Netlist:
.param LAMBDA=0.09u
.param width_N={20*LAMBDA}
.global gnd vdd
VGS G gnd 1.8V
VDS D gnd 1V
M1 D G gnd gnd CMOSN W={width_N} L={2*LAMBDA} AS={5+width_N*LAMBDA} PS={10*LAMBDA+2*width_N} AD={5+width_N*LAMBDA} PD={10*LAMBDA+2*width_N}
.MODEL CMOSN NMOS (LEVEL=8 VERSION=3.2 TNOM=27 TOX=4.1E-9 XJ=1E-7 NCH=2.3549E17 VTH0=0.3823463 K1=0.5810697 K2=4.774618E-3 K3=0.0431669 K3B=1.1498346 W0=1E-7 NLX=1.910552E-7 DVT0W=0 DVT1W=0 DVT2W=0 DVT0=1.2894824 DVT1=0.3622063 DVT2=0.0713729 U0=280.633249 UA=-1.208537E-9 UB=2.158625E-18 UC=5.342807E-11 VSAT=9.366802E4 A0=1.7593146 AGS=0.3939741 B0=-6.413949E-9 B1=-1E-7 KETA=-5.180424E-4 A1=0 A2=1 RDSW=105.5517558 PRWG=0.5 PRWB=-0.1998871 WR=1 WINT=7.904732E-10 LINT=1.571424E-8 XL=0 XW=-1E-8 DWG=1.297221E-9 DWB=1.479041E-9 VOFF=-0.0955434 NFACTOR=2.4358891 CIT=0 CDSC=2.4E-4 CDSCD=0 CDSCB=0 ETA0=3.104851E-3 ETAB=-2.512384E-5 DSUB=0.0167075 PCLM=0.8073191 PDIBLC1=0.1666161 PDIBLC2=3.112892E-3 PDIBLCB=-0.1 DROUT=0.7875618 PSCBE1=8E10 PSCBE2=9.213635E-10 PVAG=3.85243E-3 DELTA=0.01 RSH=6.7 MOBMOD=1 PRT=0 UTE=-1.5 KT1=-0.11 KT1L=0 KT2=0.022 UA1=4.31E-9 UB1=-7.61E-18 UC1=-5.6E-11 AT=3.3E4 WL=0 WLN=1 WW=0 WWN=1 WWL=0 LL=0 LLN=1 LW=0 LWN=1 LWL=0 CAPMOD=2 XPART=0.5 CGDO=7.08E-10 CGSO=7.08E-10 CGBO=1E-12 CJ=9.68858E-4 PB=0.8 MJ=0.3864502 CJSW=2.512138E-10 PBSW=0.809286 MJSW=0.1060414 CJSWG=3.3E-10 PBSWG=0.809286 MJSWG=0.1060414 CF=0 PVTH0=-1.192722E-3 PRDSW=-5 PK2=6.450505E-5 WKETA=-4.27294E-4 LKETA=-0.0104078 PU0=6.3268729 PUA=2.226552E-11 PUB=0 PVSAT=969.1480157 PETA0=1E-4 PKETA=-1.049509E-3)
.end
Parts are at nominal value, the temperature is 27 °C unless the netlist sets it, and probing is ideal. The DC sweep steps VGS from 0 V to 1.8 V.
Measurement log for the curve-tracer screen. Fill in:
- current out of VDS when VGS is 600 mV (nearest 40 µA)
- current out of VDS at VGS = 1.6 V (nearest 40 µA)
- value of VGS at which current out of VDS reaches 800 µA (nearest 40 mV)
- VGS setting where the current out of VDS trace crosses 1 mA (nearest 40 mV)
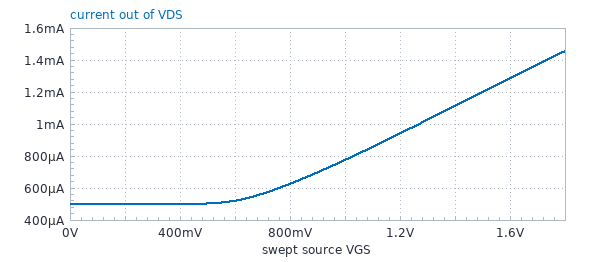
520 µA
1.28 mA
1.04 V
1.28 V
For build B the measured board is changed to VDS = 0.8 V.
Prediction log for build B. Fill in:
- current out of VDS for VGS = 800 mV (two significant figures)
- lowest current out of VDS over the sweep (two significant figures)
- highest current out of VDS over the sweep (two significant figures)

620 µA
500 µA
1.4 mA
